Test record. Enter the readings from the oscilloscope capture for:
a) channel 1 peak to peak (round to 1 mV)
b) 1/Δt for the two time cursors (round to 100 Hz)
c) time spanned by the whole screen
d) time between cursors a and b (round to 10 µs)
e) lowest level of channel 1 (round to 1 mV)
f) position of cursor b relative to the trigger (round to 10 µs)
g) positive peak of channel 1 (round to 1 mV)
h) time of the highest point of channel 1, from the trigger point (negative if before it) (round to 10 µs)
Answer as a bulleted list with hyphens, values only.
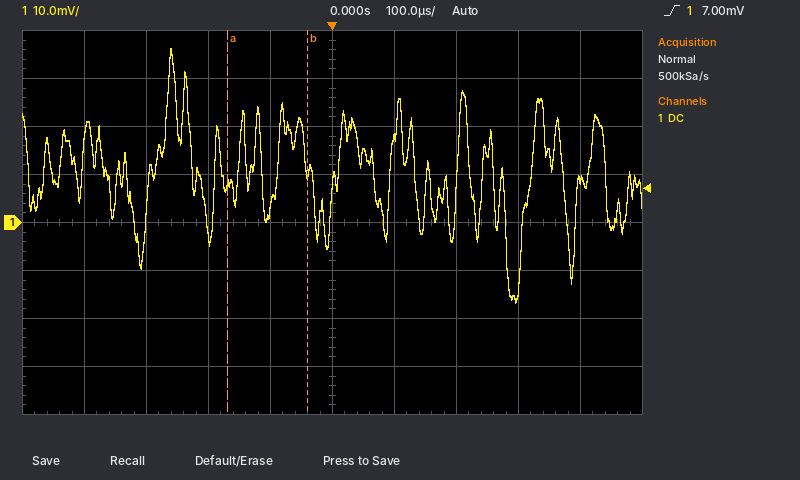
- 53 mV
- 7.7 kHz
- 1 ms
- 130 µs
- -17 mV
- -40 µs
- 36 mV
- -260 µs
